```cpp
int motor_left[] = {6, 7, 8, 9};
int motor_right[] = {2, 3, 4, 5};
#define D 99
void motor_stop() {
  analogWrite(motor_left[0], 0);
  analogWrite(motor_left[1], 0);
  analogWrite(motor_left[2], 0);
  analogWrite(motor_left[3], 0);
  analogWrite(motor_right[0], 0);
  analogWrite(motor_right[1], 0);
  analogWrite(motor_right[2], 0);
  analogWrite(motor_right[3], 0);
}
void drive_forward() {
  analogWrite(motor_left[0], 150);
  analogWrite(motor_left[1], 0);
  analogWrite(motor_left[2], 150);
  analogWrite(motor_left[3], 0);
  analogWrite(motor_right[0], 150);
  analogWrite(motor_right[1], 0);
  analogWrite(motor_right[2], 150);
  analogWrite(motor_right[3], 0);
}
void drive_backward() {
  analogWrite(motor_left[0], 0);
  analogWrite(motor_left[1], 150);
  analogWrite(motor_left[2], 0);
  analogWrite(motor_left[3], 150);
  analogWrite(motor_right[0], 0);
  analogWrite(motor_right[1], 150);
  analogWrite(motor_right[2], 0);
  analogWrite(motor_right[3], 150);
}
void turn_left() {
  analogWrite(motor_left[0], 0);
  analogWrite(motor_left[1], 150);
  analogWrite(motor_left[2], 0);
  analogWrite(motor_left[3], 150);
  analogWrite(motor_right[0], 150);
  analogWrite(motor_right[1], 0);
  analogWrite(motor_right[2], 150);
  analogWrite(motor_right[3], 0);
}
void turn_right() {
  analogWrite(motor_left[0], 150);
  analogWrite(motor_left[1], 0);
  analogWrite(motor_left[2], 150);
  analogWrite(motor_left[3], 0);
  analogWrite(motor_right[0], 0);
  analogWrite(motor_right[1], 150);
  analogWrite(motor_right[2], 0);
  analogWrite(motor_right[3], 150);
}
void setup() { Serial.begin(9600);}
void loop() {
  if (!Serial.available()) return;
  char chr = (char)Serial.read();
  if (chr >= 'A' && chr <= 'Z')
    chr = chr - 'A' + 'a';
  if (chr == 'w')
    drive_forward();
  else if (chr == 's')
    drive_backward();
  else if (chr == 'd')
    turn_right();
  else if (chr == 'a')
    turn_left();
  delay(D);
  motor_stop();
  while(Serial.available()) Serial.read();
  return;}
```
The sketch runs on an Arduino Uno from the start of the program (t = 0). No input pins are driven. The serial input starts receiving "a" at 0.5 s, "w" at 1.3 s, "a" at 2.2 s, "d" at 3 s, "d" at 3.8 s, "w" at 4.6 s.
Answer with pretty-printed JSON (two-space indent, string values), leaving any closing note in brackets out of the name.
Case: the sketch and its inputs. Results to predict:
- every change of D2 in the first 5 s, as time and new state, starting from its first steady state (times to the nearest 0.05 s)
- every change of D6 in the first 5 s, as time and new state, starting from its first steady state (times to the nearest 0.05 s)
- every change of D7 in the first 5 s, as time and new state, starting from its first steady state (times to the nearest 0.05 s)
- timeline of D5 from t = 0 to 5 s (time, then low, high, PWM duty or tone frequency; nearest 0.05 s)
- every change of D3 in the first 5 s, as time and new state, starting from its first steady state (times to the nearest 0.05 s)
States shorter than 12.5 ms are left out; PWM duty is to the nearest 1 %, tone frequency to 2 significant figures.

{
  "every change of D2 in the first 5 s, as time and new state, starting from its first steady state": "0.5 s high; 0.6 s low; 1.3 s high; 1.4 s low; 2.2 s high; 2.3 s low; 4.6 s high; 4.7 s low",
  "every change of D6 in the first 5 s, as time and new state, starting from its first steady state": "0.5 s low; 1.3 s PWM 59 %; 1.4 s low; 3 s PWM 59 %; 3.1 s low; 3.8 s PWM 59 %; 3.9 s low; 4.6 s PWM 59 %; 4.7 s low",
  "every change of D7 in the first 5 s, as time and new state, starting from its first steady state": "0.5 s high; 0.6 s low; 2.2 s high; 2.3 s low",
  "timeline of D5 from t = 0 to 5 s": "0.5 s low; 3 s PWM 59 %; 3.1 s low; 3.8 s PWM 59 %; 3.9 s low",
  "every change of D3 in the first 5 s, as time and new state, starting from its first steady state": "0.5 s low; 3 s PWM 59 %; 3.1 s low; 3.8 s PWM 59 %; 3.9 s low"
}
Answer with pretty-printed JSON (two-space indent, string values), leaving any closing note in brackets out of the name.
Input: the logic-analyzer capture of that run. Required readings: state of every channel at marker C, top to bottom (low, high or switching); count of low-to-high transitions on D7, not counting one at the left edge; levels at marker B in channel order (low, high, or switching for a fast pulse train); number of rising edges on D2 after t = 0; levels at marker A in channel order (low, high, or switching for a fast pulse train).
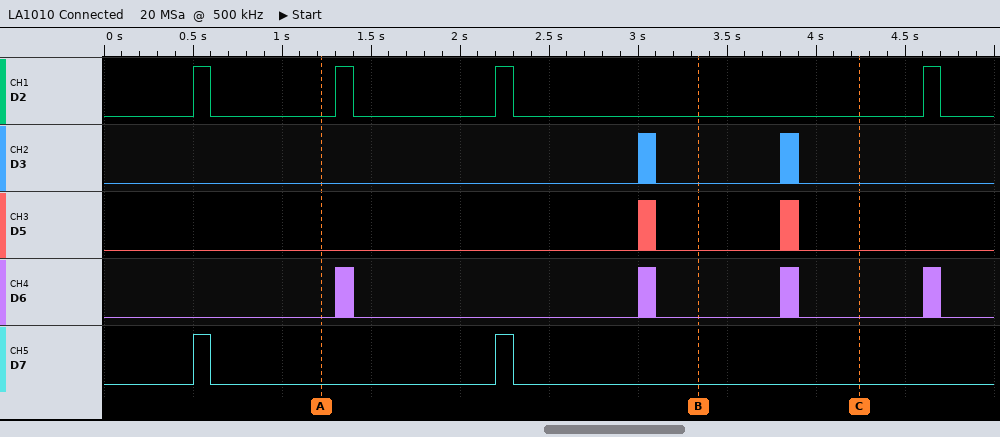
{
  "state of every channel at marker C, top to bottom": "D2 low, D3 low, D5 low, D6 low, D7 low",
  "count of low-to-high transitions on D7, not counting one at the left edge": "2",
  "levels at marker B in channel order": "D2 low, D3 low, D5 low, D6 low, D7 low",
  "number of rising edges on D2 after t = 0": "4",
  "levels at marker A in channel order": "D2 low, D3 low, D5 low, D6 low, D7 low"
}
